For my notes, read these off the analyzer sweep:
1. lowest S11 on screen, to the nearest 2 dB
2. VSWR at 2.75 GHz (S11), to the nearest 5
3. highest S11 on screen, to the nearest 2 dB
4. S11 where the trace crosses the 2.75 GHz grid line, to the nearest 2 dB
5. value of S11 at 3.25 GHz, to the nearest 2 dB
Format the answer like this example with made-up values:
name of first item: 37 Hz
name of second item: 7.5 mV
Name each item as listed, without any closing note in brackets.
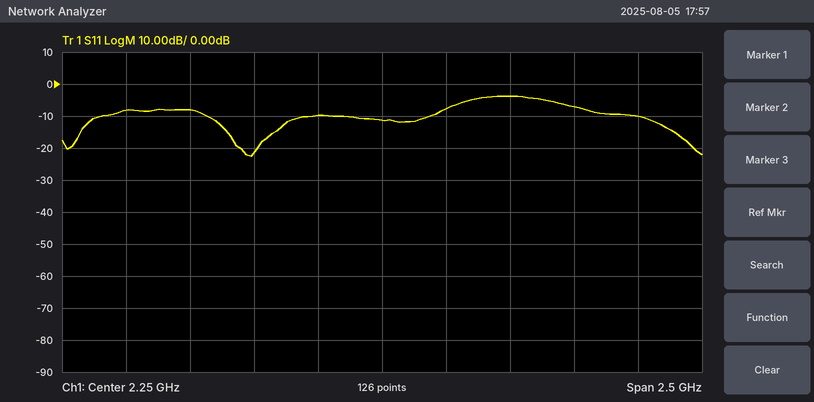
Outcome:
lowest S11 on screen, to the nearest 2 dB: -22 dB
VSWR at 2.75 GHz (S11), to the nearest 5: 5
highest S11 on screen, to the nearest 2 dB: -4 dB
S11 where the trace crosses the 2.75 GHz grid line, to the nearest 2 dB: -4 dB
value of S11 at 3.25 GHz, to the nearest 2 dB: -10 dB
